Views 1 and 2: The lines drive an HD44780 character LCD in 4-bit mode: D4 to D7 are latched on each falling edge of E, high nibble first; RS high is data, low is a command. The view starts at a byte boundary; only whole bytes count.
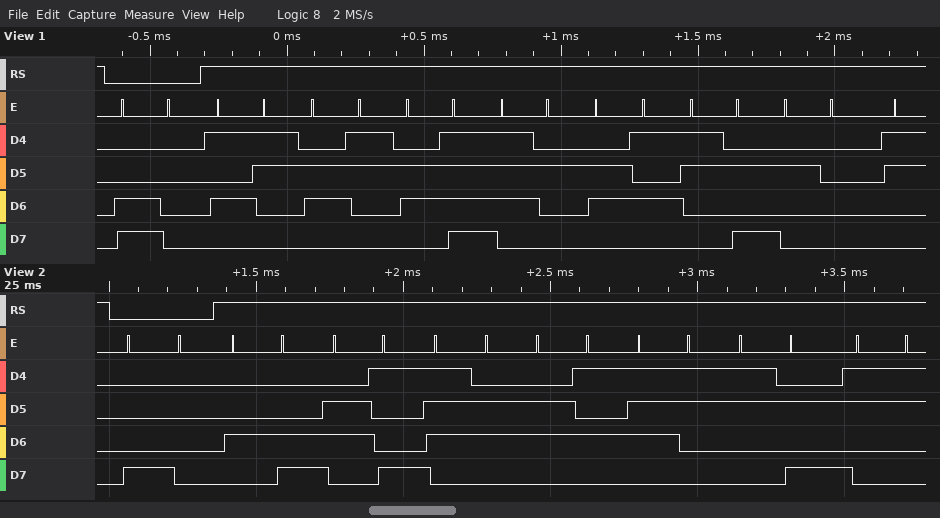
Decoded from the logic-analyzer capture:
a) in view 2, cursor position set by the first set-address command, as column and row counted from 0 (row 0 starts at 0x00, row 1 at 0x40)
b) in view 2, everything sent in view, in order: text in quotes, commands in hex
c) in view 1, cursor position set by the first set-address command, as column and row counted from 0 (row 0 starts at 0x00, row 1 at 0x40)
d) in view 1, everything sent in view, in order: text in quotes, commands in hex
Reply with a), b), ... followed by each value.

a) column 0, row 0
b) 0x80 "Lives:3"
c) column 0, row 1
d) 0xC0 "Score: "
